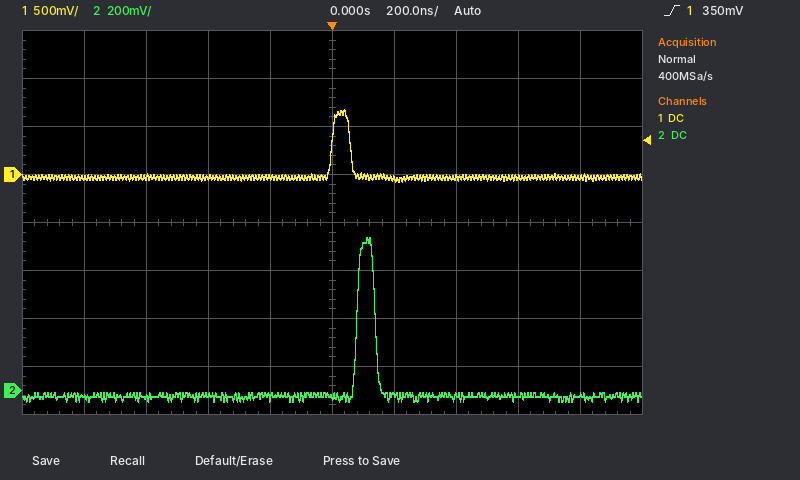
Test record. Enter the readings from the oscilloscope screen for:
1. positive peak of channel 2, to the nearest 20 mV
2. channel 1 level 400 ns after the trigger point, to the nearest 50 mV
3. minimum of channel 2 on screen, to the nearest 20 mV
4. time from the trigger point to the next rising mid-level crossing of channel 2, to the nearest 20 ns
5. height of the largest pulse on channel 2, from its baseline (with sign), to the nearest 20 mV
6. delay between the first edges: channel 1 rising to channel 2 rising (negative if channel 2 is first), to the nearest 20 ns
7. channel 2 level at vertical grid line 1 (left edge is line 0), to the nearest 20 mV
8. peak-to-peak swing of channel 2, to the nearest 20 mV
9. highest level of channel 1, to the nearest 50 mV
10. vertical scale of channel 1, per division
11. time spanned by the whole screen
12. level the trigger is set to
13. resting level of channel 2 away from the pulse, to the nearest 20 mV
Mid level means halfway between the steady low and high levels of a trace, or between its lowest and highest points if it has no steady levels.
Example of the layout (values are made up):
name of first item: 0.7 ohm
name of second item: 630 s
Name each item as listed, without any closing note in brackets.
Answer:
positive peak of channel 2, to the nearest 20 mV: 640 mV
channel 1 level 400 ns after the trigger point, to the nearest 50 mV: -50 mV
minimum of channel 2 on screen, to the nearest 20 mV: -40 mV
time from the trigger point to the next rising mid-level crossing of channel 2, to the nearest 20 ns: 80 ns
height of the largest pulse on channel 2, from its baseline (with sign), to the nearest 20 mV: +660 mV
delay between the first edges: channel 1 rising to channel 2 rising (negative if channel 2 is first), to the nearest 20 ns: +80 ns
channel 2 level at vertical grid line 1 (left edge is line 0), to the nearest 20 mV: -20 mV
peak-to-peak swing of channel 2, to the nearest 20 mV: 680 mV
highest level of channel 1, to the nearest 50 mV: 700 mV
vertical scale of channel 1, per division: 500 mV
time spanned by the whole screen: 2 µs
level the trigger is set to: 350 mV
resting level of channel 2 away from the pulse, to the nearest 20 mV: -20 mV
